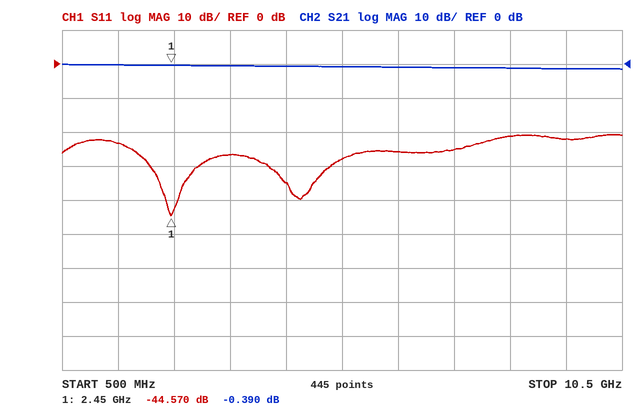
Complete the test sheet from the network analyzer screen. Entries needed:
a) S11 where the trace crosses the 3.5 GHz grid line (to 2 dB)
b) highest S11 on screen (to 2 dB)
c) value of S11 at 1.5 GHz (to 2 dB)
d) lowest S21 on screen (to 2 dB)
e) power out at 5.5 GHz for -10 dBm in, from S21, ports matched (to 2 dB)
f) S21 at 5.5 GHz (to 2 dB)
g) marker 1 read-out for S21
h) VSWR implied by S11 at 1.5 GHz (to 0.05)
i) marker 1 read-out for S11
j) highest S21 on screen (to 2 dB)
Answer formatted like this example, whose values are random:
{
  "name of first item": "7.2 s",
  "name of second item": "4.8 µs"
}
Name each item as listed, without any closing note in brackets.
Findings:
{
  "S11 where the trace crosses the 3.5 GHz grid line": "-26 dB",
  "highest S11 on screen": "-20 dB",
  "value of S11 at 1.5 GHz": "-24 dB",
  "lowest S21 on screen": "-2 dB",
  "power out at 5.5 GHz for -10 dBm in, from S21, ports matched": "-10 dBm",
  "S21 at 5.5 GHz": "0 dB",
  "marker 1 read-out for S21": "-0.390 dB",
  "VSWR implied by S11 at 1.5 GHz": "1.15",
  "marker 1 read-out for S11": "-44.570 dB",
  "highest S21 on screen": "0 dB"
}
